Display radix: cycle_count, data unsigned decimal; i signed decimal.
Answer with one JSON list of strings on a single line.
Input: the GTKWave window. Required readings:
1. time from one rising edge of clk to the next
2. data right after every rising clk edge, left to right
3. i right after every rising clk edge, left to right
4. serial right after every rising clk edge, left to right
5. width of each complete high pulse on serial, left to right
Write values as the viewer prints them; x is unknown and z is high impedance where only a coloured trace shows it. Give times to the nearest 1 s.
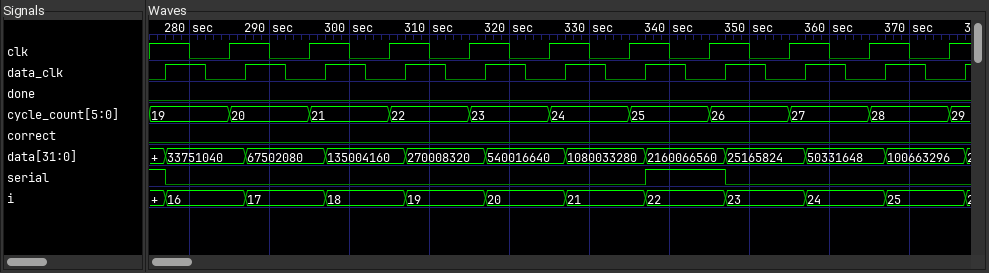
["10 s", "33751040, 67502080, 135004160, 270008320, 540016640, 1080033280, 2160066560, 25165824, 50331648, 100663296", "16, 17, 18, 19, 20, 21, 22, 23, 24, 25", "0 0 0 0 0 0 1 0 0 0", "10 s"]
